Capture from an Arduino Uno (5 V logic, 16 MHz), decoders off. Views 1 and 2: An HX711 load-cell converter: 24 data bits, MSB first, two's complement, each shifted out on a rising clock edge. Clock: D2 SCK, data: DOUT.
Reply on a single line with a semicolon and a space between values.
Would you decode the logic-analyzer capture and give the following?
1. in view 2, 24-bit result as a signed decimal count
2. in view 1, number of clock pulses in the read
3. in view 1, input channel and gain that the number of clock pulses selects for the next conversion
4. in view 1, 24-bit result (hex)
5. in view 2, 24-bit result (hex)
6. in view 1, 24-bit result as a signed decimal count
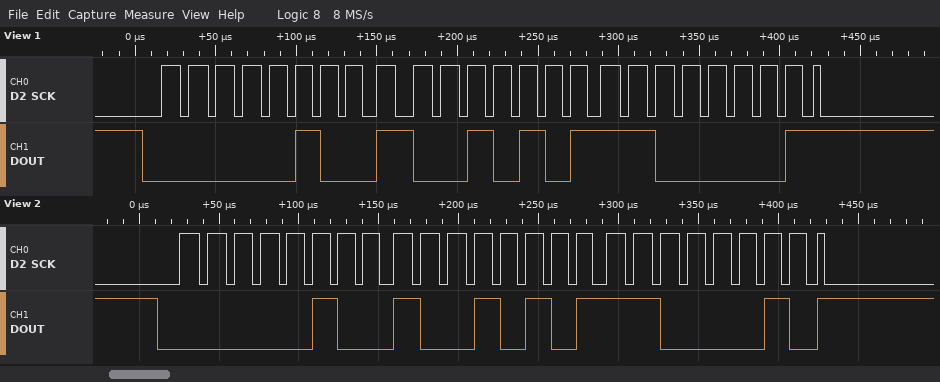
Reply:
300482; 25; channel A, gain 128; 0x0495C1; 0x0495C2; 300481
